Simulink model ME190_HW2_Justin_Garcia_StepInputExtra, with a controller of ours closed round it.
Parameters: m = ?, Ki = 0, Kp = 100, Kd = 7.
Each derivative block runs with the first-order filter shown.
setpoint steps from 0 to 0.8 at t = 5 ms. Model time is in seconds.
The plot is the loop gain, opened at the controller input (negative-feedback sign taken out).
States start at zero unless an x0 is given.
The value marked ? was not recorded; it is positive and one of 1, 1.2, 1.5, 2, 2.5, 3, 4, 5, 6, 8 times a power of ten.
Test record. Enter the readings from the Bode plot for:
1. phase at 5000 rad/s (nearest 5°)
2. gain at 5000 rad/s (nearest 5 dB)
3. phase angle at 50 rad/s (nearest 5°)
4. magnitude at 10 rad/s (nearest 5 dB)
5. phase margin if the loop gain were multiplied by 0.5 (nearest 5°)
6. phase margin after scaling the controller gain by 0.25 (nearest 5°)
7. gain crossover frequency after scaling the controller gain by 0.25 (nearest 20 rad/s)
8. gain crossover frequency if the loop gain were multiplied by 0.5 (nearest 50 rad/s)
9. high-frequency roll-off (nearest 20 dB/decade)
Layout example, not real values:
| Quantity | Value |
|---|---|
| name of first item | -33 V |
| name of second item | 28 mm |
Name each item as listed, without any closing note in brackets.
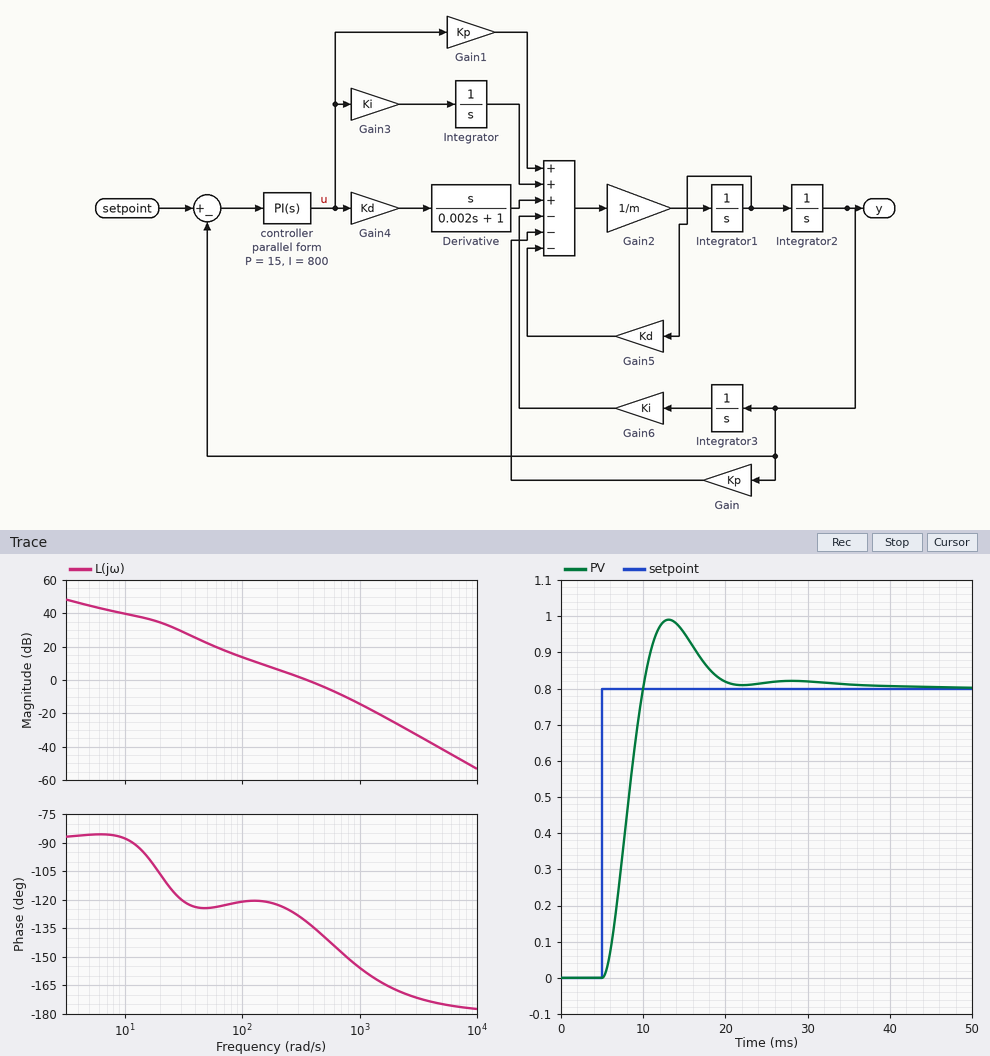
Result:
| Quantity | Value |
|---|---|
| phase at 5000 rad/s | -175° |
| gain at 5000 rad/s | -40 dB |
| phase angle at 50 rad/s | -125° |
| magnitude at 10 rad/s | 40 dB |
| phase margin if the loop gain were multiplied by 0.5 | 55° |
| phase margin after scaling the controller gain by 0.25 | 60° |
| gain crossover frequency after scaling the controller gain by 0.25 | 120 rad/s |
| gain crossover frequency if the loop gain were multiplied by 0.5 | 200 rad/s |
| high-frequency roll-off | -40 dB/decade |
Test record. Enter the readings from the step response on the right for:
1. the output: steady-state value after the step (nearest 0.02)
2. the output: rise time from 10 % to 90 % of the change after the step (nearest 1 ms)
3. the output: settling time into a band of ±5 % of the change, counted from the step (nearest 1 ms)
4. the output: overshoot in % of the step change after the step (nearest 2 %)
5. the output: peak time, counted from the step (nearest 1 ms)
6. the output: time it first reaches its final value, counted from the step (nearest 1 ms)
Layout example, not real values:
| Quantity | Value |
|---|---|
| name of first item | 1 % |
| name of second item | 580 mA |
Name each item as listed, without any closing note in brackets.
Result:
| Quantity | Value |
|---|---|
| the output: steady-state value after the step | 0.80 |
| the output: rise time from 10 % to 90 % of the change after the step | 3 ms |
| the output: settling time into a band of ±5 % of the change, counted from the step | 14 ms |
| the output: overshoot in % of the step change after the step | 24 % |
| the output: peak time, counted from the step | 8 ms |
| the output: time it first reaches its final value, counted from the step | 5 ms |
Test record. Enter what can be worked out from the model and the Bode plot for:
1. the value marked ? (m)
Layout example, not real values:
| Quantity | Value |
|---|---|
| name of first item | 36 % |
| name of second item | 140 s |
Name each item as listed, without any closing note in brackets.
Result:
| Quantity | Value |
|---|---|
| the value marked ? | 0.25 |
